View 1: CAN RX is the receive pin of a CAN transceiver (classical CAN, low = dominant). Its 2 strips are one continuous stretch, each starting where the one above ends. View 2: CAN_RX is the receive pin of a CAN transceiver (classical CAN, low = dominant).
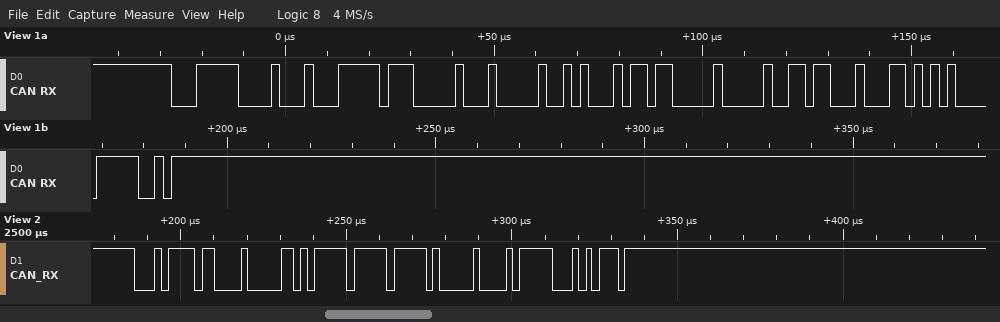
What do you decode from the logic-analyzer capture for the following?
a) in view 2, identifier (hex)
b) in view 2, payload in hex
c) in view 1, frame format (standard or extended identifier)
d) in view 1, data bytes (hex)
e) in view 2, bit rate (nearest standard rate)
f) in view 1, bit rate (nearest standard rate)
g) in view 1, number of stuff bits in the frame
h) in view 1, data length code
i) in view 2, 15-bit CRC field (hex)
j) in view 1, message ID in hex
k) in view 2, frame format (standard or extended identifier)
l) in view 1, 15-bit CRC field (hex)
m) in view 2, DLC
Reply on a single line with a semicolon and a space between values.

0x17B; 15 FF FE 00; standard; FF 00 80 A2 D8 00 6C 46; 500 kbit/s; 500 kbit/s; 7; 8; 0x5F2B; 0x1F1; standard; 0x543E; 4
